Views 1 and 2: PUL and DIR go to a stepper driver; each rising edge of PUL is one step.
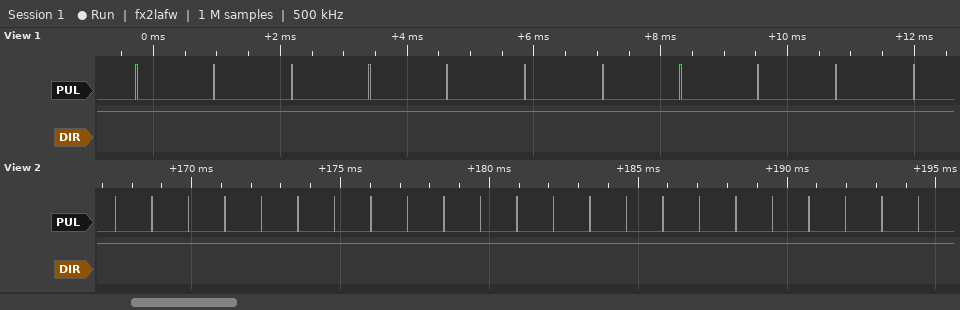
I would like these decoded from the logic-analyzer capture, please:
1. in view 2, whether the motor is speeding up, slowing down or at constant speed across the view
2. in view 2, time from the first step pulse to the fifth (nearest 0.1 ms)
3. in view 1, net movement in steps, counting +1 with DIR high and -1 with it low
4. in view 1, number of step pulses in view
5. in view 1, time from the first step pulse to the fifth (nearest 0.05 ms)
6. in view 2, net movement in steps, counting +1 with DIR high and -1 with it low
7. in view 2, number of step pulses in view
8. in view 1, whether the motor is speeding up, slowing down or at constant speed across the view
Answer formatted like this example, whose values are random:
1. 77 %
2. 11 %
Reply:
1. constant speed
2. 4.9 ms
3. +11
4. 11
5. 4.90 ms
6. +23
7. 23
8. constant speed
